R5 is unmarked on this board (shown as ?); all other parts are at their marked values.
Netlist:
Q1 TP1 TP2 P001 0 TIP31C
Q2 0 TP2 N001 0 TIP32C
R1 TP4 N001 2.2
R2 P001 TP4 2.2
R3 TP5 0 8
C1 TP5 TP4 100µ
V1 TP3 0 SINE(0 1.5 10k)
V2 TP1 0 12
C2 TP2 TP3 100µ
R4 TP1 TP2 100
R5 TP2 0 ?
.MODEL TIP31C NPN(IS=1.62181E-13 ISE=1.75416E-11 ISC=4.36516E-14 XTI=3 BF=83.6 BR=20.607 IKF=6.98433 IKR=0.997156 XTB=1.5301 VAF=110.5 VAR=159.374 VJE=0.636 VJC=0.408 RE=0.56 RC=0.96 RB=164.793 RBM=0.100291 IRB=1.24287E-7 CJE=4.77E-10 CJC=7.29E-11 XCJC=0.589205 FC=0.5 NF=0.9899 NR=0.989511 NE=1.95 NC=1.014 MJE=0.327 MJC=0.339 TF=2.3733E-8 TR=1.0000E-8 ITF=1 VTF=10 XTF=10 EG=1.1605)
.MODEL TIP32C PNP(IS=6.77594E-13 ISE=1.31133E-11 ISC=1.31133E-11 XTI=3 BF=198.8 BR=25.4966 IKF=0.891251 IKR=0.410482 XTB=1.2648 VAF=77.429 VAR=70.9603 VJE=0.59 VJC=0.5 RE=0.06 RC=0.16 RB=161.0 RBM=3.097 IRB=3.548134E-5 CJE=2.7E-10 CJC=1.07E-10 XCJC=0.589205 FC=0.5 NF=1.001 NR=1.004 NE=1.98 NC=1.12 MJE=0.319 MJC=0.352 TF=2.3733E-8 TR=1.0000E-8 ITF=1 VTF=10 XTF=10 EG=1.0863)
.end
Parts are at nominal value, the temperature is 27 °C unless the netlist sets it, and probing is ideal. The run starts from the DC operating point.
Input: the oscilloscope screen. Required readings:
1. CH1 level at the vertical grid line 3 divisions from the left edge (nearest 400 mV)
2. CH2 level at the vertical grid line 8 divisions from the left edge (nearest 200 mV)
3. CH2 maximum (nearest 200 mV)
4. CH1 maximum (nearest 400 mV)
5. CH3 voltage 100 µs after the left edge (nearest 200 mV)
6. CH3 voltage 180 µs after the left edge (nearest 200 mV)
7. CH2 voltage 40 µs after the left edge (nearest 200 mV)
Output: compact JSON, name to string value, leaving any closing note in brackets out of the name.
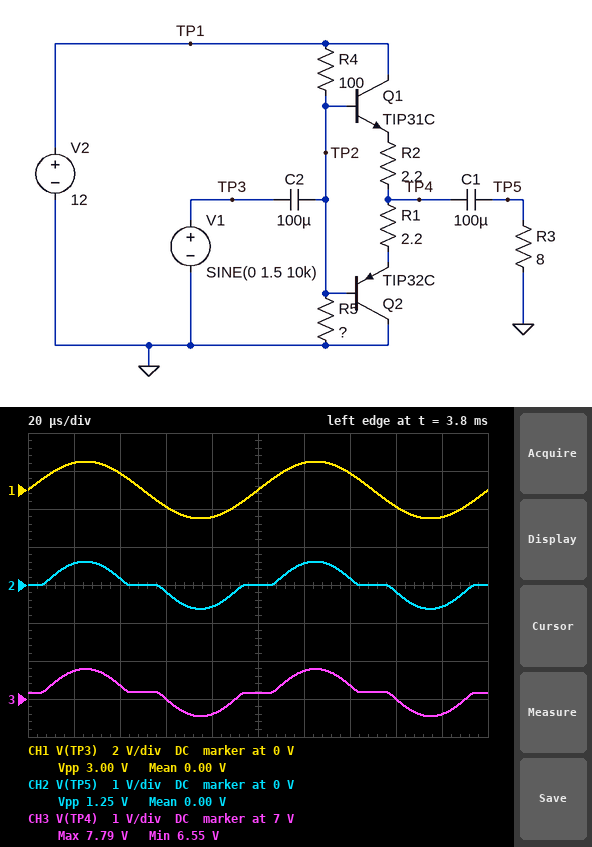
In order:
{"CH1 level at the vertical grid line 3 divisions from the left edge": "-800 mV", "CH2 level at the vertical grid line 8 divisions from the left edge": "-200 mV", "CH2 maximum": "600 mV", "CH1 maximum": "1.6 V", "CH3 voltage 100 µs after the left edge": "7.2 V", "CH3 voltage 180 µs after the left edge": "6.6 V", "CH2 voltage 40 µs after the left edge": "200 mV"}
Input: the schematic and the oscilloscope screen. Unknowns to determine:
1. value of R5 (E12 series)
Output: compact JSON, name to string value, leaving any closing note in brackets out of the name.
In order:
{"value of R5": "150 Ω"}
